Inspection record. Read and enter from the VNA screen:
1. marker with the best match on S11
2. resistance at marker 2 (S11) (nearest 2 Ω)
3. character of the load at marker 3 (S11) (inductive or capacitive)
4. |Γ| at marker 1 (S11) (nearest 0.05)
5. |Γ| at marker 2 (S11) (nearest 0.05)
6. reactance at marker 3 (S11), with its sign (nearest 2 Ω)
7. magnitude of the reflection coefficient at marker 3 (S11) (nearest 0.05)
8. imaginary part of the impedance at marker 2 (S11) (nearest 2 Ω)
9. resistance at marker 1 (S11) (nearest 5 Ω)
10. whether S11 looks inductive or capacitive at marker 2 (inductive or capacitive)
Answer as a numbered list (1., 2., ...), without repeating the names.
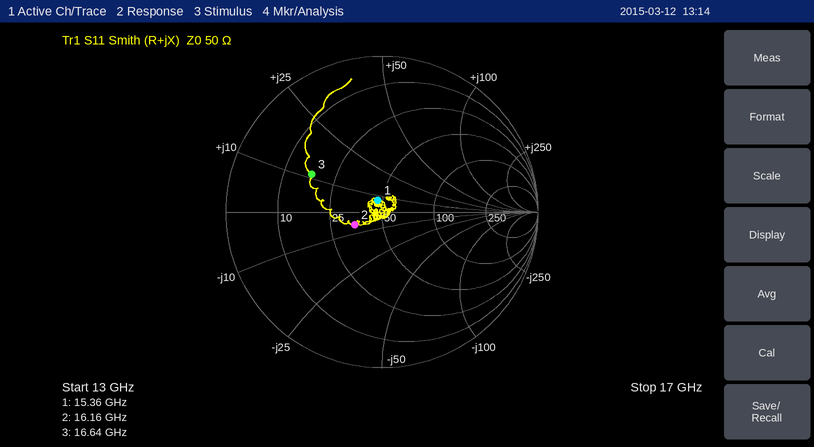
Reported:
1. marker 1
2. 34 Ω
3. inductive
4. 0.10
5. 0.20
6. +12 Ω
7. 0.50
8. -6 Ω
9. 45 Ω
10. capacitive
